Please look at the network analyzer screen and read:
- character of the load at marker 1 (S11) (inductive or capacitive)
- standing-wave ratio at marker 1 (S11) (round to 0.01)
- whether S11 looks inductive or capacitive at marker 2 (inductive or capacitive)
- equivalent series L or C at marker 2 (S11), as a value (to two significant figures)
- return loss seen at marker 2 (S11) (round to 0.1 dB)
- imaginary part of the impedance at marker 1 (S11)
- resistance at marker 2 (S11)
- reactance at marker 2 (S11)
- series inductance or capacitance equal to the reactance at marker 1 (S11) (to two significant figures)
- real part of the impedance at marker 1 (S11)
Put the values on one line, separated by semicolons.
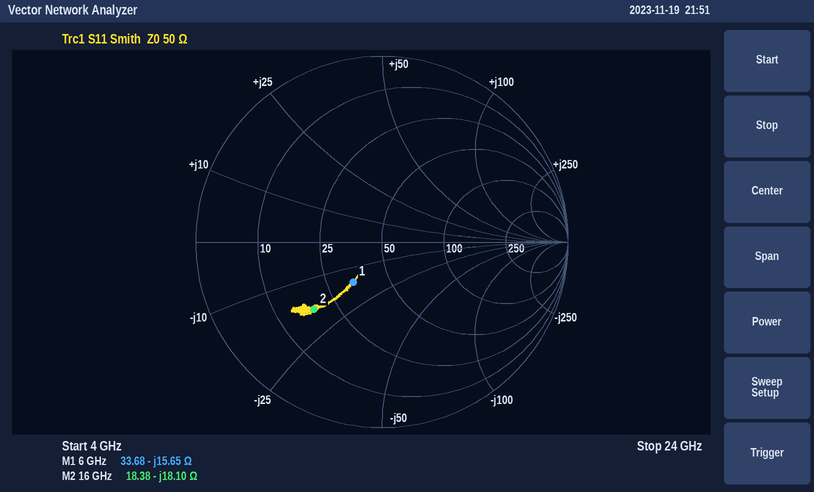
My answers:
capacitive; 1.72; capacitive; 550 fF; 5.8 dB; -15.65 Ω; 18.38 Ω; -18.10 Ω; 1.7 pF; 33.68 Ω
